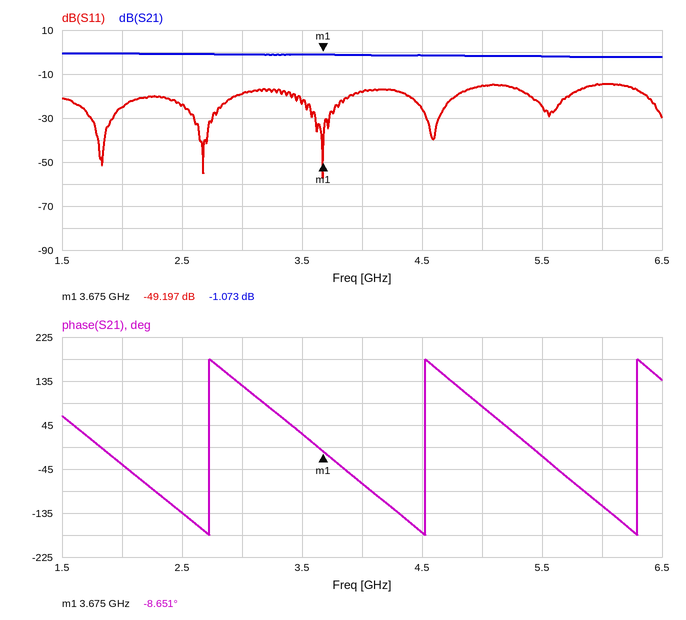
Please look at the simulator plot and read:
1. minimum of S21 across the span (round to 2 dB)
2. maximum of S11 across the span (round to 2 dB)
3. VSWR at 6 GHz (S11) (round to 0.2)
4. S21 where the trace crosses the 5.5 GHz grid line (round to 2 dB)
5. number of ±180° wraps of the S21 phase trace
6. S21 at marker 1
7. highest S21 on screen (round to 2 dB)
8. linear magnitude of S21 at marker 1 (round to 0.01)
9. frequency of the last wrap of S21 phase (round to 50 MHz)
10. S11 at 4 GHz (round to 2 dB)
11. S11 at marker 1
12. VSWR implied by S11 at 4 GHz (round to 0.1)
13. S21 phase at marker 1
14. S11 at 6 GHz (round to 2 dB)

-2 dB
-14 dB
1.4
-2 dB
3
-1.073 dB
0 dB
0.88
6.30 GHz
-18 dB
-49.197 dB
1.3
-8.651°
-14 dB
